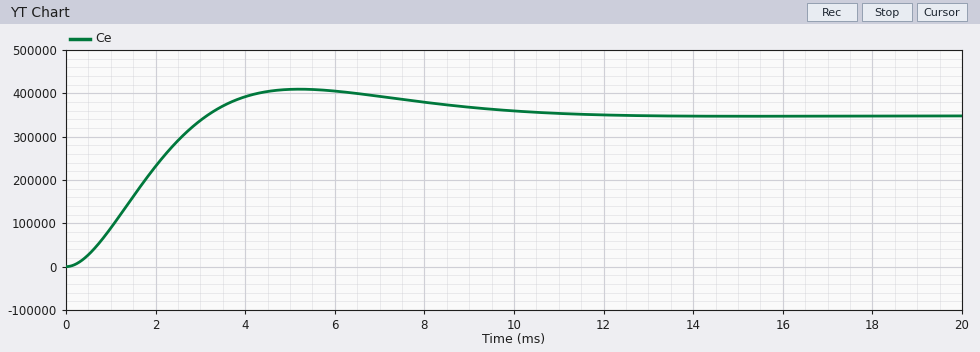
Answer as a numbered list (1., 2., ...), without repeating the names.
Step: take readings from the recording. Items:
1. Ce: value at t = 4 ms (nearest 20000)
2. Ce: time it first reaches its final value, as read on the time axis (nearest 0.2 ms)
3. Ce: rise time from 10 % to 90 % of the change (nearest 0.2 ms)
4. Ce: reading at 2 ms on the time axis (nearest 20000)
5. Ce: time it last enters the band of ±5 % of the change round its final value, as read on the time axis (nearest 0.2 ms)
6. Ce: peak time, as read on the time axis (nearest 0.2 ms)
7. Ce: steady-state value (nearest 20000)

1. 400000
2. 3.2 ms
3. 2.2 ms
4. 240000
5. 9.2 ms
6. 5.2 ms
7. 340000
